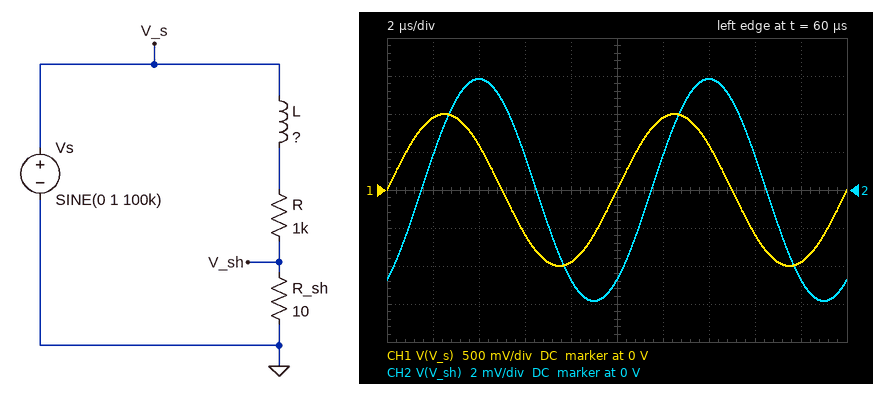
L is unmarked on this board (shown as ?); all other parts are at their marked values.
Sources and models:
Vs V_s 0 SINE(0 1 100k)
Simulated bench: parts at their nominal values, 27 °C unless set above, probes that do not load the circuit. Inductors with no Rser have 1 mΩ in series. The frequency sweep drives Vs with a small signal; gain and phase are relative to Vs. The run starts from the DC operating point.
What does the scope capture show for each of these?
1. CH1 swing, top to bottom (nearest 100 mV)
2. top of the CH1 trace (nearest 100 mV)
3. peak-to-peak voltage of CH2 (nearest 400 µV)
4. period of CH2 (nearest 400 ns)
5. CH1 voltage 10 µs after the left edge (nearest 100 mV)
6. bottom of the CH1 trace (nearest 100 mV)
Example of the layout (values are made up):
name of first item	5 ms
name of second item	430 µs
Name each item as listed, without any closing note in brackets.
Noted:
CH1 swing, top to bottom	2.0 V
top of the CH1 trace	1.0 V
peak-to-peak voltage of CH2	11.6 mV
period of CH2	10.0 µs
CH1 voltage 10 µs after the left edge	0 V
bottom of the CH1 trace	-1.0 V
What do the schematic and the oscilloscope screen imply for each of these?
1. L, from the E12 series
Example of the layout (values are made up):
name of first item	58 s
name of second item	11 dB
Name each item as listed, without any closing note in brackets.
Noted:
L, from the E12 series	2.2 mH
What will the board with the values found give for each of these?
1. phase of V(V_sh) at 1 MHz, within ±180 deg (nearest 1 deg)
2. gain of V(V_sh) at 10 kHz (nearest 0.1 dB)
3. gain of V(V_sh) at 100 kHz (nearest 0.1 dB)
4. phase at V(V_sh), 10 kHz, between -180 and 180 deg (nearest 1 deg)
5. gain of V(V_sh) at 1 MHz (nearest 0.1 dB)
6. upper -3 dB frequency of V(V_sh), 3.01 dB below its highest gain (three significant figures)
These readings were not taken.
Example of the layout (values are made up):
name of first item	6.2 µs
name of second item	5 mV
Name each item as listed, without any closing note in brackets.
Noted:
phase of V(V_sh) at 1 MHz, within ±180 deg	-86 deg
gain of V(V_sh) at 10 kHz	-40.2 dB
gain of V(V_sh) at 100 kHz	-44.7 dB
phase at V(V_sh), 10 kHz, between -180 and 180 deg	-8 deg
gain of V(V_sh) at 1 MHz	-62.8 dB
upper -3 dB frequency of V(V_sh), 3.01 dB below its highest gain	73.1 kHz
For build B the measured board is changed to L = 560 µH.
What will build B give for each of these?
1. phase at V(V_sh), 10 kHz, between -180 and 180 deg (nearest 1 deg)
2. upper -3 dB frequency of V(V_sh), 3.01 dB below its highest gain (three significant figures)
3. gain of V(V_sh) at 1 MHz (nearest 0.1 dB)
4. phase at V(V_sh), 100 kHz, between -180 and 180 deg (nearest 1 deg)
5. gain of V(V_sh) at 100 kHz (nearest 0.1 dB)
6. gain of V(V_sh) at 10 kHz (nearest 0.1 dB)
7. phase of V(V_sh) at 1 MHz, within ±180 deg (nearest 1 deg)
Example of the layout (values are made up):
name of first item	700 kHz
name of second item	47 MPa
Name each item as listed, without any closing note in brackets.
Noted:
phase at V(V_sh), 10 kHz, between -180 and 180 deg	-2 deg
upper -3 dB frequency of V(V_sh), 3.01 dB below its highest gain	287 kHz
gain of V(V_sh) at 1 MHz	-51.3 dB
phase at V(V_sh), 100 kHz, between -180 and 180 deg	-19 deg
gain of V(V_sh) at 100 kHz	-40.6 dB
gain of V(V_sh) at 10 kHz	-40.1 dB
phase of V(V_sh) at 1 MHz, within ±180 deg	-74 deg
